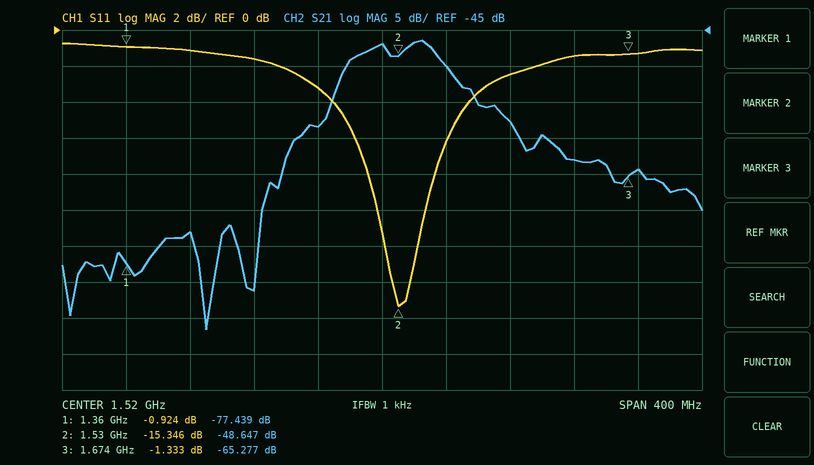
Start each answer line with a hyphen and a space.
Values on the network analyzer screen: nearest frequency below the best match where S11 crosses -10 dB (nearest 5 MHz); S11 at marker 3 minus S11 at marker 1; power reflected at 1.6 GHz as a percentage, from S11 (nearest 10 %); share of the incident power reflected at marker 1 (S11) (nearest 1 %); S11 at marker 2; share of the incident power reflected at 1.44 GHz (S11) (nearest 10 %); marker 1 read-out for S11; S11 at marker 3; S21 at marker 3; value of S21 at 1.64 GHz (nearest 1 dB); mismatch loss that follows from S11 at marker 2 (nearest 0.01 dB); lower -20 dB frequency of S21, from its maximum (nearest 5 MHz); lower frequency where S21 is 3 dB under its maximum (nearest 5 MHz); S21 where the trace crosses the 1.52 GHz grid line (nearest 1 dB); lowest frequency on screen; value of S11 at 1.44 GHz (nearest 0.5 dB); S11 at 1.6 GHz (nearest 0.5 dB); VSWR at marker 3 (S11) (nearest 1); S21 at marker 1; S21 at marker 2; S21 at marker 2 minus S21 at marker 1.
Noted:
- 1.515 GHz
- -0.409 dB
- 60 %
- 81 %
- -15.346 dB
- 70 %
- -0.924 dB
- -1.333 dB
- -65.277 dB
- -63 dB
- 0.13 dB
- 1.455 GHz
- 1.500 GHz
- -47 dB
- 1.32 GHz
- -1.5 dB
- -2.5 dB
- 13
- -77.439 dB
- -48.647 dB
- 28.792 dB
